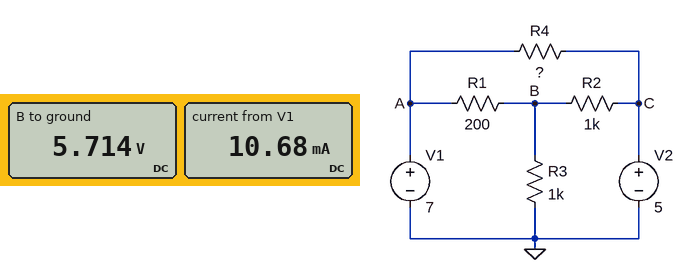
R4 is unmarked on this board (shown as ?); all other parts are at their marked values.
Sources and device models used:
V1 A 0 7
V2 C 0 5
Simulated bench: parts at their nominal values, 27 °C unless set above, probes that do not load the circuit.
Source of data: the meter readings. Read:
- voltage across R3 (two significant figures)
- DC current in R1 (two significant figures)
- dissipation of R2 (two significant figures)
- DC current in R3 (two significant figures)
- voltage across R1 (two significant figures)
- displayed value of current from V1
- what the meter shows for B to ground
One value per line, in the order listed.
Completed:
5.7 V
6.4 mA
510 µW
5.7 mA
1.3 V
10.68 mA
5.714 V
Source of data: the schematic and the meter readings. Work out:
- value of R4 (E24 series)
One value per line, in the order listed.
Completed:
470 Ω
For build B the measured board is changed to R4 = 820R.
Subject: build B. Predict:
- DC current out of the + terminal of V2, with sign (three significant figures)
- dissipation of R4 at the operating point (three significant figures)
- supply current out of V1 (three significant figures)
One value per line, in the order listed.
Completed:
-3.15 mA
4.88 mW
8.87 mA
